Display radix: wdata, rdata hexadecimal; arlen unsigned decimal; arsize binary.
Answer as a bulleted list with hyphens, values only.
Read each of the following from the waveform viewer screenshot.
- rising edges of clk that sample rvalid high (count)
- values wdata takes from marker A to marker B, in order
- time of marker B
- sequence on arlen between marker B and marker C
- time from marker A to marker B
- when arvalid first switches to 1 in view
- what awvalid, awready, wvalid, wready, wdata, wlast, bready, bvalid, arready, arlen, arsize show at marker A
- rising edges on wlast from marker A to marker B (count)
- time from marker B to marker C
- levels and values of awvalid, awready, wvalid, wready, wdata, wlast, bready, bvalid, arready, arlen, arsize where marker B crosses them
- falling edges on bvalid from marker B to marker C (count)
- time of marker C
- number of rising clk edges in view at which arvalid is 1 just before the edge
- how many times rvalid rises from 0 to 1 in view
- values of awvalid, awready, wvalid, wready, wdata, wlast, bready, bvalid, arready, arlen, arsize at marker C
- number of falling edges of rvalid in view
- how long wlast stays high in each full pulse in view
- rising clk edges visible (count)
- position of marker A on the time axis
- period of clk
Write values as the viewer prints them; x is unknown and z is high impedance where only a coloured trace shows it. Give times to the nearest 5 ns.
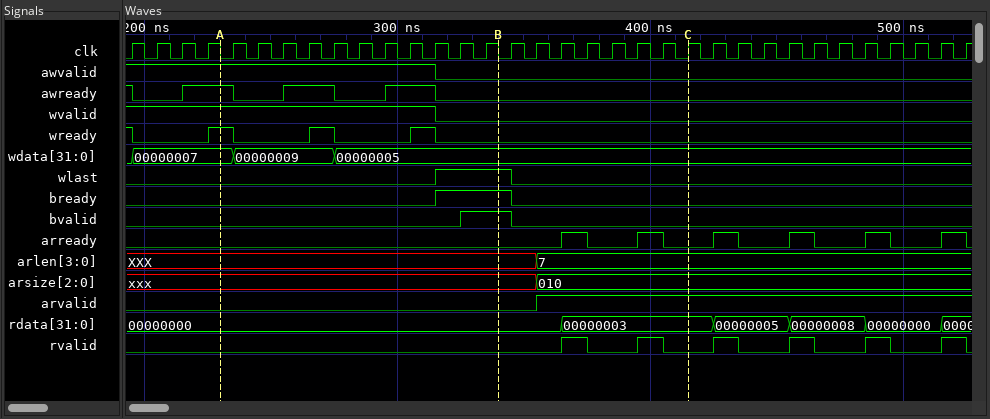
- 6
- 00000007, 00000009, 00000005
- 340 ns
- XXX, 7
- 110 ns
- 355 ns
- awvalid=1, awready=1, wvalid=1, wready=1, wdata=00000007, wlast=0, bready=0, bvalid=0, arready=0, arlen=XXX, arsize=xxx
- 1
- 75 ns
- awvalid=0, awready=0, wvalid=0, wready=0, wdata=00000005, wlast=1, bready=1, bvalid=1, arready=0, arlen=XXX, arsize=xxx
- 1
- 415 ns
- 17
- 6
- awvalid=0, awready=0, wvalid=0, wready=0, wdata=00000005, wlast=0, bready=0, bvalid=0, arready=0, arlen=7, arsize=010
- 6
- 30 ns
- 34
- 230 ns
- 10 ns
